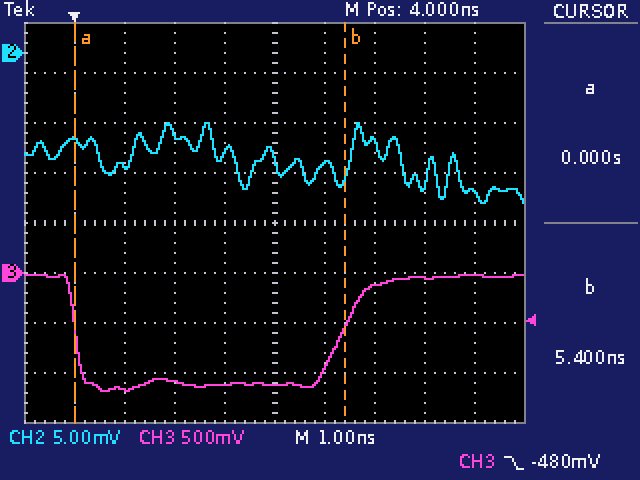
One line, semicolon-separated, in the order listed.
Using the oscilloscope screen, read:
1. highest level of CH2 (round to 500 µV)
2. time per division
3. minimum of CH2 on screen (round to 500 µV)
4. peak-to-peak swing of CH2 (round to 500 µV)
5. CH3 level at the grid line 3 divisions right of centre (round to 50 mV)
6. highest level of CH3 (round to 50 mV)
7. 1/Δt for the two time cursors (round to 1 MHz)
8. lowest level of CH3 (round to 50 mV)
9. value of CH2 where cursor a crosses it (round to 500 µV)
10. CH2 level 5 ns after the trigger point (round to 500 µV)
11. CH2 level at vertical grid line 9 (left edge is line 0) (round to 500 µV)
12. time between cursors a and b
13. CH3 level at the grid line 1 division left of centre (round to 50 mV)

-7.0 mV; 1 ns; -15.0 mV; 8.0 mV; -50 mV; 0 mV; 185 MHz; -1.20 V; -9.0 mV; -11.0 mV; -14.0 mV; 5.4 ns; -1.10 V
